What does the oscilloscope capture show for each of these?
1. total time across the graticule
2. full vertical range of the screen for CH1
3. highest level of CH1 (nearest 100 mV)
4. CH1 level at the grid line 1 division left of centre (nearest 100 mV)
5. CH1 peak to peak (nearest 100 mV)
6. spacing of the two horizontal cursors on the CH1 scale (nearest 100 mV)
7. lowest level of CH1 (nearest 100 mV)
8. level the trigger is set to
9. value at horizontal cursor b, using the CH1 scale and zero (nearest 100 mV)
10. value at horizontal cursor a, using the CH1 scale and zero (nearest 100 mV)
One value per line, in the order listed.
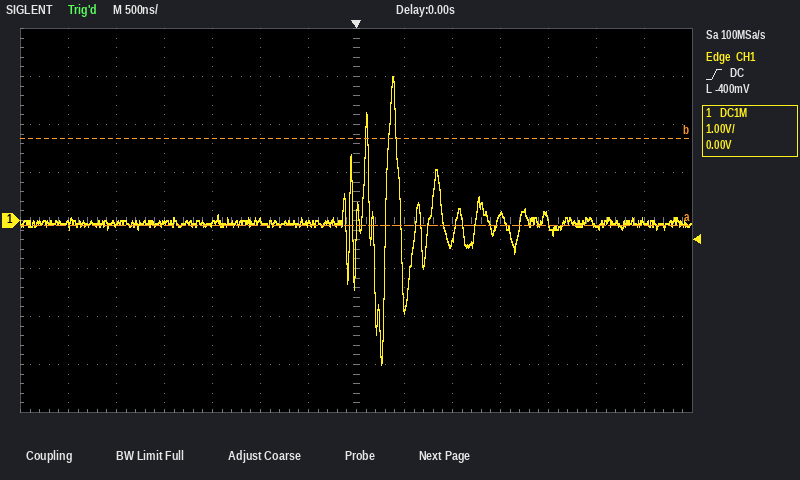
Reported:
7 µs
8 V
3.0 V
-100 mV
6.0 V
1.8 V
-3.0 V
-400 mV
1.7 V
-100 mV
